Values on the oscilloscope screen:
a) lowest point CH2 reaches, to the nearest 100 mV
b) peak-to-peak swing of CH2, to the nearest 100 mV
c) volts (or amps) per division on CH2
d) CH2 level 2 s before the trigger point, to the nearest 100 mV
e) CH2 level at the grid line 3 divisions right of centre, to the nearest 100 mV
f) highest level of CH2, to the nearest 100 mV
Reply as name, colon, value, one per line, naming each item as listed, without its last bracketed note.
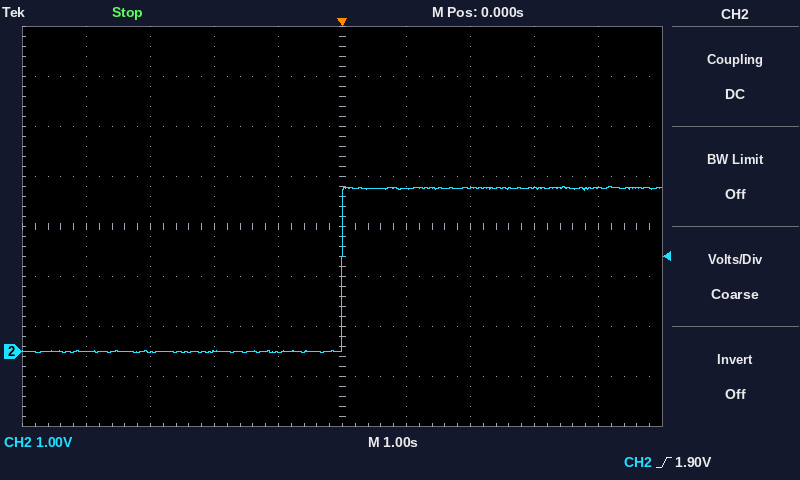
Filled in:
lowest point CH2 reaches, to the nearest 100 mV: 0.0 V
peak-to-peak swing of CH2, to the nearest 100 mV: 3.3 V
volts (or amps) per division on CH2: 1 V
CH2 level 2 s before the trigger point, to the nearest 100 mV: 0.0 V
CH2 level at the grid line 3 divisions right of centre, to the nearest 100 mV: 3.3 V
highest level of CH2, to the nearest 100 mV: 3.3 V
